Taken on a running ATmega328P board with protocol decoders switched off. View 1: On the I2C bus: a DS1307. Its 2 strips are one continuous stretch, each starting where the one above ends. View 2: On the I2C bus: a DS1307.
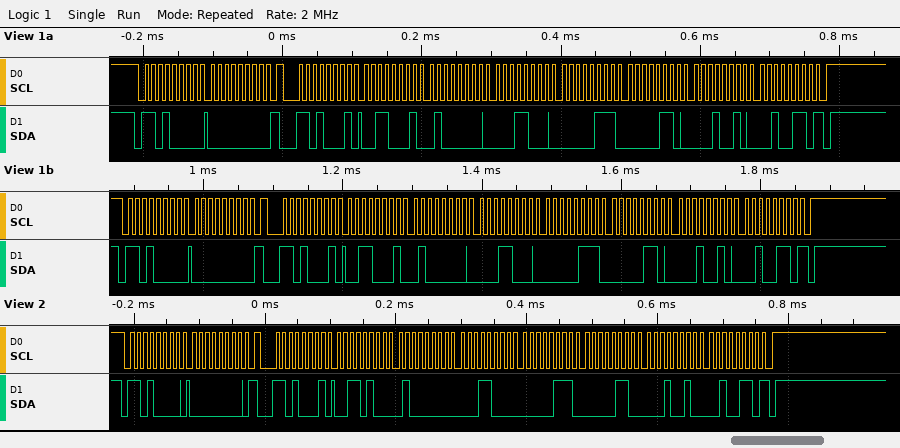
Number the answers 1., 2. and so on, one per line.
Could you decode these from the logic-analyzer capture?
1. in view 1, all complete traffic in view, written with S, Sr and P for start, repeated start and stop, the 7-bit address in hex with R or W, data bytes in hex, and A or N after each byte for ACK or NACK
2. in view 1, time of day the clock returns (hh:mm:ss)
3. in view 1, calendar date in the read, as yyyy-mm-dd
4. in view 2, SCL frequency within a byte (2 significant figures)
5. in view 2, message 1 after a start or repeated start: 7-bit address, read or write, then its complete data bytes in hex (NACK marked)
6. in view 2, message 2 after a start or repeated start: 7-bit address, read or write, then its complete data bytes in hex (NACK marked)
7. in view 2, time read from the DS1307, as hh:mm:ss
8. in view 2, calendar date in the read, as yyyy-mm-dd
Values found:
1. S 68W A 00 A Sr 68R A 31 A 40 A 18 A 07 A 06 A 12 A 26 N P S 68W A 00 A Sr 68R A 31 A 40 A 18 A 07 A 06 A 12 A 26 N P
2. 18:40:31
3. 2026-12-06
4. 100 kHz
5. 0x68 write: 00
6. 0x68 read: 34 40 18 07 06 12 26 NACK
7. 18:40:34
8. 2026-12-06
